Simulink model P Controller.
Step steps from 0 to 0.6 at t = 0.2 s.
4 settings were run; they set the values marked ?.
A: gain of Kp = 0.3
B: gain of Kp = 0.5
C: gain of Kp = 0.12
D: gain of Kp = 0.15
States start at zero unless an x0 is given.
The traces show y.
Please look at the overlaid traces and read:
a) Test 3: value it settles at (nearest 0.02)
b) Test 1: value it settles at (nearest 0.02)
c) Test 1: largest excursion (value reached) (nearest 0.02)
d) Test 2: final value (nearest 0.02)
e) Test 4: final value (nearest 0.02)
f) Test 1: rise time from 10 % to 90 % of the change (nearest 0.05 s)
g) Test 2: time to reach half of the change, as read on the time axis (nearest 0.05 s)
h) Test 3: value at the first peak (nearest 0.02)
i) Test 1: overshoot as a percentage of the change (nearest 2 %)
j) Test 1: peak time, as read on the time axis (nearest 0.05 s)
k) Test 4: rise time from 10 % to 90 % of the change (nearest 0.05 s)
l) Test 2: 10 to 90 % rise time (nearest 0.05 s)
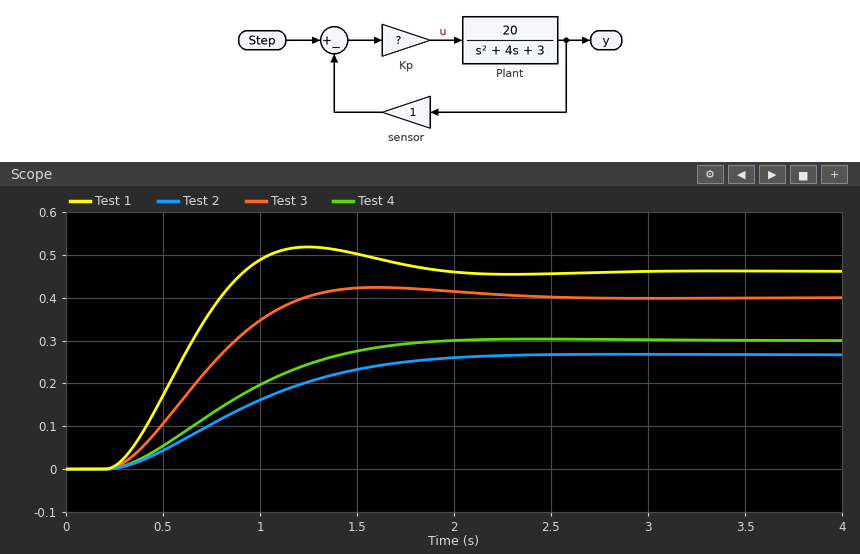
0.40
0.46
0.52
0.26
0.30
0.50 s
0.85 s
0.42
12 %
1.25 s
1.05 s
1.15 s
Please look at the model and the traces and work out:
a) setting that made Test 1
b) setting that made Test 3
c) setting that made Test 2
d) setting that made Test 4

B
A
C
D
